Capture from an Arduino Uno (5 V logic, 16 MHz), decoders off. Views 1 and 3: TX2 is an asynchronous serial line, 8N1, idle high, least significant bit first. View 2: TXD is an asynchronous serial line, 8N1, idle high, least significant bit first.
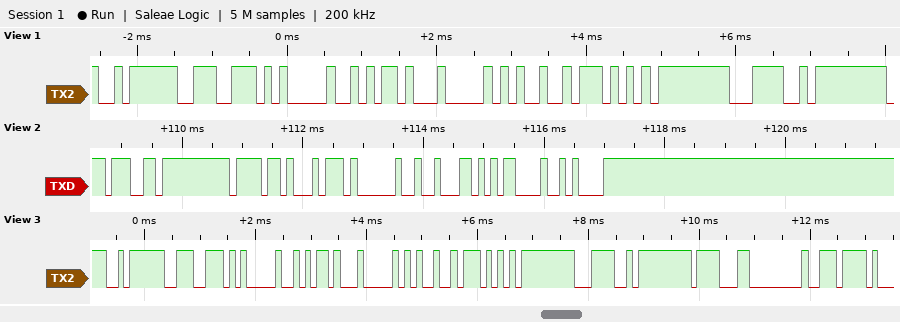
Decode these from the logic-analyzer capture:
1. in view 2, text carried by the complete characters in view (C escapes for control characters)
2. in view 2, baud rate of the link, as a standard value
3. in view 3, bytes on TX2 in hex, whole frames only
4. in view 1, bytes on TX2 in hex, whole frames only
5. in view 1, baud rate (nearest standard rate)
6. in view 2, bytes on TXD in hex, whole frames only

"got b\r\n"
9600 baud
FA CE 05 6A 04 25 57 FF 3C FF 8F 00 EE
FA CE 05 6A 04 25 57 FF 3C FF
9600 baud
67 6F 74 20 62 0D 0A
